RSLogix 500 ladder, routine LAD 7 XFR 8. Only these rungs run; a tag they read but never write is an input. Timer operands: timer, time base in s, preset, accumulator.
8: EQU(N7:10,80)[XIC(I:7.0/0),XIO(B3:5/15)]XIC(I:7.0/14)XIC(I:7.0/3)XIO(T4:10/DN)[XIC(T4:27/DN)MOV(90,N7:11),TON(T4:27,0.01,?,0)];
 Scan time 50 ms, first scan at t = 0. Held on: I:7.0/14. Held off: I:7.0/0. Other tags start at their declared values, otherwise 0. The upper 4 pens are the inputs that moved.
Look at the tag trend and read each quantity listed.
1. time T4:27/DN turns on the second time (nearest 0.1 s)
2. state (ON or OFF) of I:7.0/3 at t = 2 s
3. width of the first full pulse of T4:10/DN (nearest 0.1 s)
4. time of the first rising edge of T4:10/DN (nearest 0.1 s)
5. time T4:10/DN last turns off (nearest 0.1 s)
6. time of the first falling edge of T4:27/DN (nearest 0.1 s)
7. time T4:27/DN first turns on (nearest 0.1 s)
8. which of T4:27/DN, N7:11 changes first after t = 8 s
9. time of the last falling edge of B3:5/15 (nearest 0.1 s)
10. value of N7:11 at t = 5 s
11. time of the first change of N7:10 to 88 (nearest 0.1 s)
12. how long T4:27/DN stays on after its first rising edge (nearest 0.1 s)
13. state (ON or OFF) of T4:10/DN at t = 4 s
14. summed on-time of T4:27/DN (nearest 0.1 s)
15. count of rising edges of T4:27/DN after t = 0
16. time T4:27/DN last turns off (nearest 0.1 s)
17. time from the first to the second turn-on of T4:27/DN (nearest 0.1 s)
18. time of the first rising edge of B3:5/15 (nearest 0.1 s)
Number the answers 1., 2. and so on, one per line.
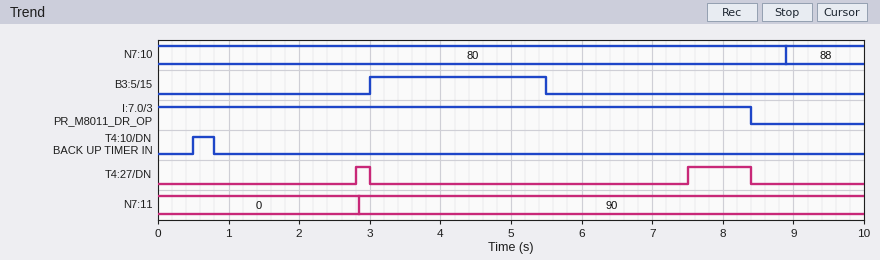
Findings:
1. 7.5 s
2. ON
3. 0.3 s
4. 0.5 s
5. 0.8 s
6. 3.0 s
7. 2.8 s
8. T4:27/DN
9. 5.5 s
10. 90
11. 8.9 s
12. 0.2 s
13. OFF
14. 1.1 s
15. 2
16. 8.4 s
17. 4.7 s
18. 3.0 s
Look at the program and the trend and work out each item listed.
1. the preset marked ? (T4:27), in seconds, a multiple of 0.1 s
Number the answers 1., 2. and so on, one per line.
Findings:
1. 2.0 s
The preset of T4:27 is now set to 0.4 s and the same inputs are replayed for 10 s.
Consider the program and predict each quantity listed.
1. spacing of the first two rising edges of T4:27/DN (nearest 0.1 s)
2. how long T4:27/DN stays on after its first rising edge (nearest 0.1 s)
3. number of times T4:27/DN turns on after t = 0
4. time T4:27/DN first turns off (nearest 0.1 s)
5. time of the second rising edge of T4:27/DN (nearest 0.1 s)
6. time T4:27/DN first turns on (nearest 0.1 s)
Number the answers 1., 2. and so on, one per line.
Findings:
1. 0.8 s
2. 0.1 s
3. 3
4. 0.5 s
5. 1.2 s
6. 0.4 s
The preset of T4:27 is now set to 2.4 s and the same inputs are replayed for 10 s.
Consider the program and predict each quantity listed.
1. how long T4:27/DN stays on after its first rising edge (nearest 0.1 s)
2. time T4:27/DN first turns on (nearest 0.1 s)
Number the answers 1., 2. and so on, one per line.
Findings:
1. 0.5 s
2. 7.9 s
